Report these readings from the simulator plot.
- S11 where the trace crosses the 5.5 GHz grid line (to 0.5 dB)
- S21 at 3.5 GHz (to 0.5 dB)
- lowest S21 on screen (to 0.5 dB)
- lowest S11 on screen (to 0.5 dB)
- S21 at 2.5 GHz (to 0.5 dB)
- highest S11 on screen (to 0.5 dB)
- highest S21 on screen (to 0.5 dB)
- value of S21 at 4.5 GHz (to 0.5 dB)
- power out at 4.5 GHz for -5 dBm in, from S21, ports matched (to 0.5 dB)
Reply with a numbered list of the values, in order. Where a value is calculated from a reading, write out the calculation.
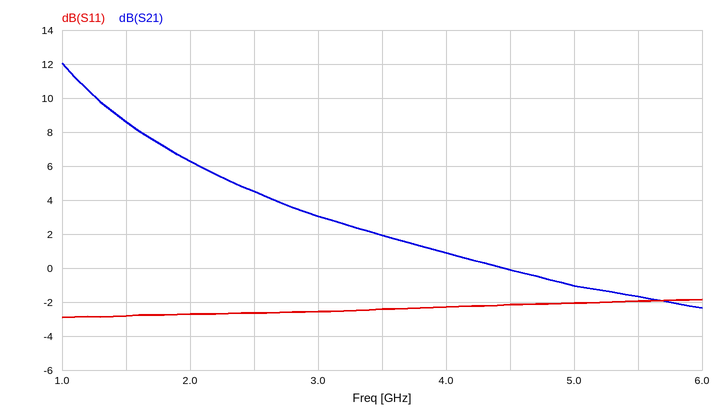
1. -2.0 dB
2. 2.0 dB
3. -2.5 dB
4. -3.0 dB
5. 4.5 dB
6. -2.0 dB
7. 12.0 dB
8. 0.0 dB
9. -5 dBm + (0.0 dB) = -5.0 dBm
